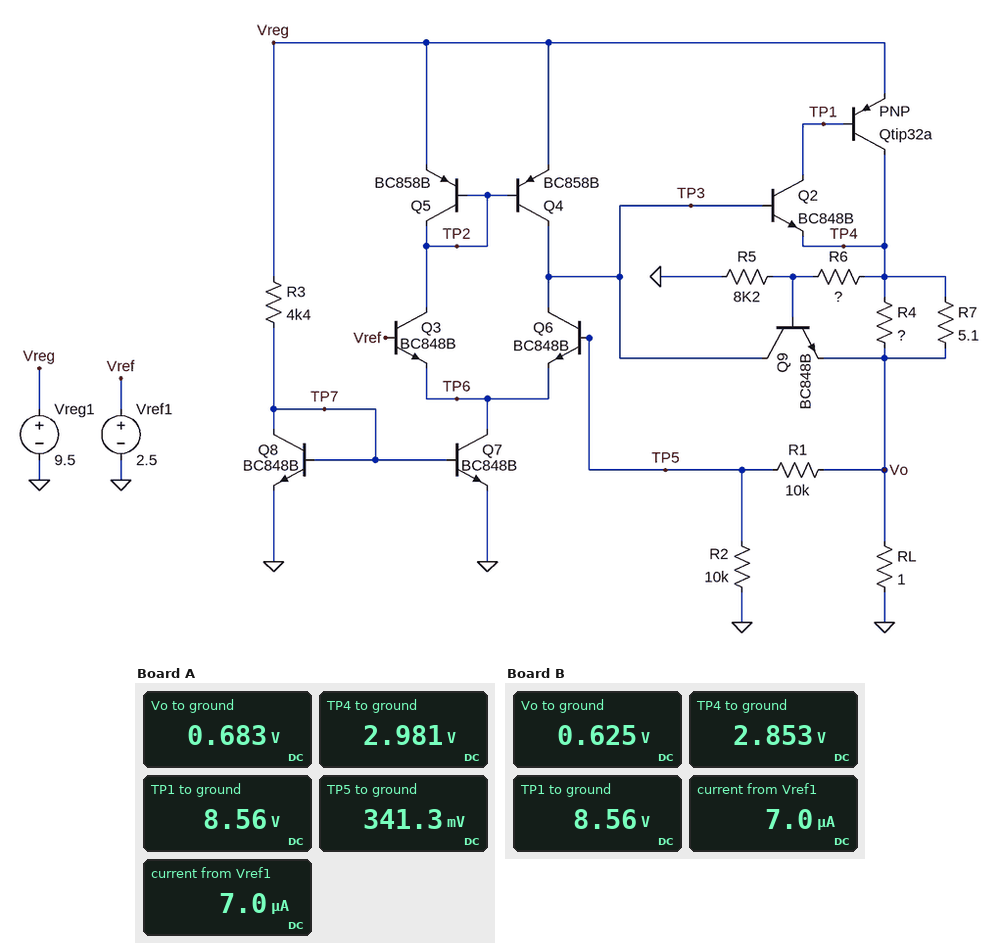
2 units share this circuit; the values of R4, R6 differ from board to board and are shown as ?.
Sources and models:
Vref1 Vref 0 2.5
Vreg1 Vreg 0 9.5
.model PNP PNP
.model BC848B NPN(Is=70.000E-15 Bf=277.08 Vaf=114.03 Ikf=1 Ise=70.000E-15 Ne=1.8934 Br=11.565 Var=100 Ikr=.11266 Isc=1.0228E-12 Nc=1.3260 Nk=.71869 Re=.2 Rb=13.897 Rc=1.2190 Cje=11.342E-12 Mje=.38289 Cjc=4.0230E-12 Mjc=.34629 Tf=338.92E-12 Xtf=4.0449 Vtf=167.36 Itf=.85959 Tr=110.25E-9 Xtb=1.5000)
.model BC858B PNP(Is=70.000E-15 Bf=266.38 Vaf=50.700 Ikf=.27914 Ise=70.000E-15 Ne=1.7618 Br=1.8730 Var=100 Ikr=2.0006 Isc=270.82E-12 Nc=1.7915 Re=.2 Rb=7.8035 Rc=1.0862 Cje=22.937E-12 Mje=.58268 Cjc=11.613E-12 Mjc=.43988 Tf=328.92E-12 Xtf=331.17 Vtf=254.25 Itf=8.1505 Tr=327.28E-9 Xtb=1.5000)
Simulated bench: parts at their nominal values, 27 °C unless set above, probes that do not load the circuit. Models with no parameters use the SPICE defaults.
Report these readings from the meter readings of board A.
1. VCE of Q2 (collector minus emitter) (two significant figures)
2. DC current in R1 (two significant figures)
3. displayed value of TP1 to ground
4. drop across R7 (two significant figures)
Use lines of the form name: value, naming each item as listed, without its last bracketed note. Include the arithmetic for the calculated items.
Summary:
VCE of Q2 (collector minus emitter): 8.56 V - 2.981 V = 5.6 V
DC current in R1: (683 mV - 341.3 mV) / 10 kΩ = 34 µA
displayed value of TP1 to ground: 8.56 V
drop across R7: 2.981 V - 683 mV = 2.3 V
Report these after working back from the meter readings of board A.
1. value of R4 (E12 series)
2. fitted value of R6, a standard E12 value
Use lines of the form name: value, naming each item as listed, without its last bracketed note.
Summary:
value of R4: 10 Ω
fitted value of R6, a standard E12 value: 10 kΩ
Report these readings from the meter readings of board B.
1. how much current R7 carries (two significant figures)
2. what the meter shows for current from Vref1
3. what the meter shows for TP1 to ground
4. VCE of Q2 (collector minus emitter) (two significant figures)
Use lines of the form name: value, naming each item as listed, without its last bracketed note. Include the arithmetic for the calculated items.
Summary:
how much current R7 carries: (2.853 V - 625 mV) / 5.1 Ω = 440 mA
what the meter shows for current from Vref1: 7.0 µA
what the meter shows for TP1 to ground: 8.56 V
VCE of Q2 (collector minus emitter): 8.56 V - 2.853 V = 5.7 V
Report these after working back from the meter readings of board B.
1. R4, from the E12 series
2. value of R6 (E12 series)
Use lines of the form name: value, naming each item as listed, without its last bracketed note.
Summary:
R4, from the E12 series: 12 Ω
value of R6: 10 kΩ
